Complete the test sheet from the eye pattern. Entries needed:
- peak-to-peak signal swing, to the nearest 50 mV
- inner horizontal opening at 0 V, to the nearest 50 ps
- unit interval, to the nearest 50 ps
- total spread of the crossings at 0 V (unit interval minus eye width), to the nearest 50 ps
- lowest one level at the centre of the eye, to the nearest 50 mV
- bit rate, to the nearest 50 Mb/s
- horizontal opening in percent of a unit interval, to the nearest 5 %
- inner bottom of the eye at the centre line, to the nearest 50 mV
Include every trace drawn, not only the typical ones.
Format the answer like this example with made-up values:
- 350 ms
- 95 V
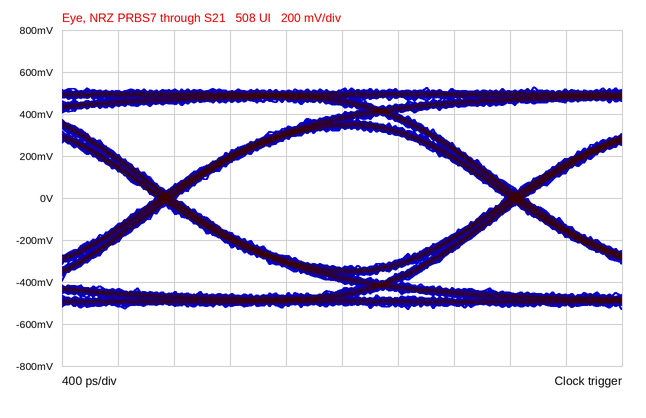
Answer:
- 1.05 V
- 2.35 ns
- 2.50 ns
- 150 ps
- 350 mV
- 400 Mb/s
- 95 %
- -350 mV
